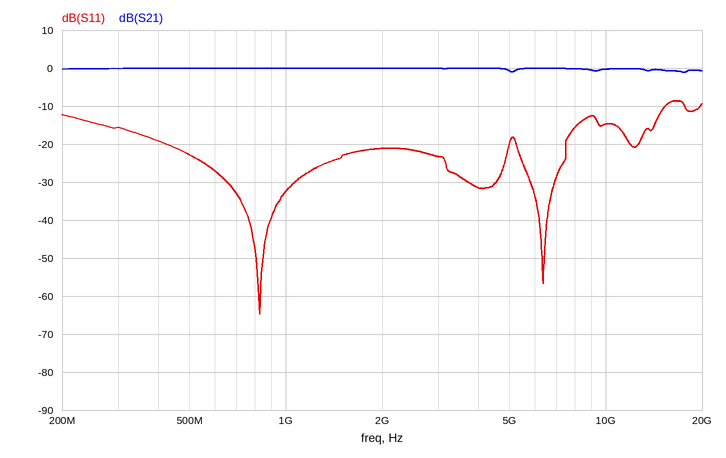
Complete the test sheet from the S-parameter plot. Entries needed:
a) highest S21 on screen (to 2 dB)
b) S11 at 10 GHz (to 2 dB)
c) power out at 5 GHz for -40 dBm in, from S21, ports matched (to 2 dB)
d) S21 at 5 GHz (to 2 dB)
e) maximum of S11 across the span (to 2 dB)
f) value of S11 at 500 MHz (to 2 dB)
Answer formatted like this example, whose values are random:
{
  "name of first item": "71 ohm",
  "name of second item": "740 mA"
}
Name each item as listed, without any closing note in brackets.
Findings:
{
  "highest S21 on screen": "0 dB",
  "S11 at 10 GHz": "-14 dB",
  "power out at 5 GHz for -40 dBm in, from S21, ports matched": "-40 dBm",
  "S21 at 5 GHz": "0 dB",
  "maximum of S11 across the span": "-8 dB",
  "value of S11 at 500 MHz": "-22 dB"
}
